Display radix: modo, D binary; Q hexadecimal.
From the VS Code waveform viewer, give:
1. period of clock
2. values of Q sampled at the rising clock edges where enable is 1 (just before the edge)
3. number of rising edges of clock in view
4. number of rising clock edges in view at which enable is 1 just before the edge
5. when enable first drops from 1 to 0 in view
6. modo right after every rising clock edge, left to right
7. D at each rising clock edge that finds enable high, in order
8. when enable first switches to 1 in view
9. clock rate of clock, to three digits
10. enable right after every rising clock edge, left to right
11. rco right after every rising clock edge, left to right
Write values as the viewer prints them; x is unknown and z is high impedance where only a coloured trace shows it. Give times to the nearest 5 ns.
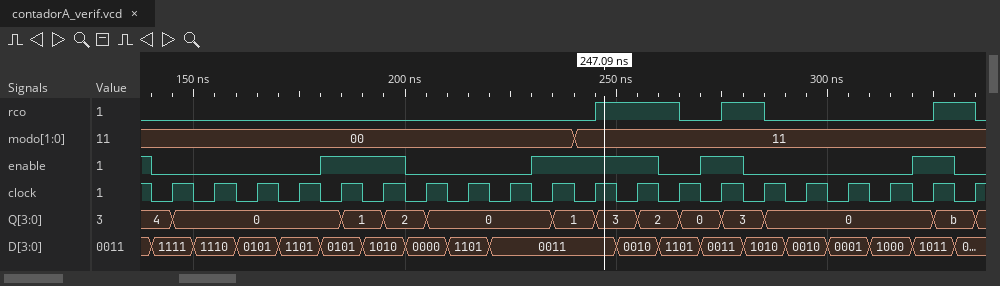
10 ns
0, 1, 0, 1, 3, 0, 0
20
7
140 ns
00, 00, 00, 00, 00, 00, 00, 00, 00, 00, 11, 11, 11, 11, 11, 11, 11, 11, 11, 11
0101, 1010, 0011, 0011, 0010, 0011, 1011
180 ns
100 MHz
0 0 0 0 1 1 0 0 0 1 1 1 0 1 0 0 0 0 1 0
0 0 0 0 0 0 0 0 0 0 1 1 0 1 0 0 0 0 1 0
